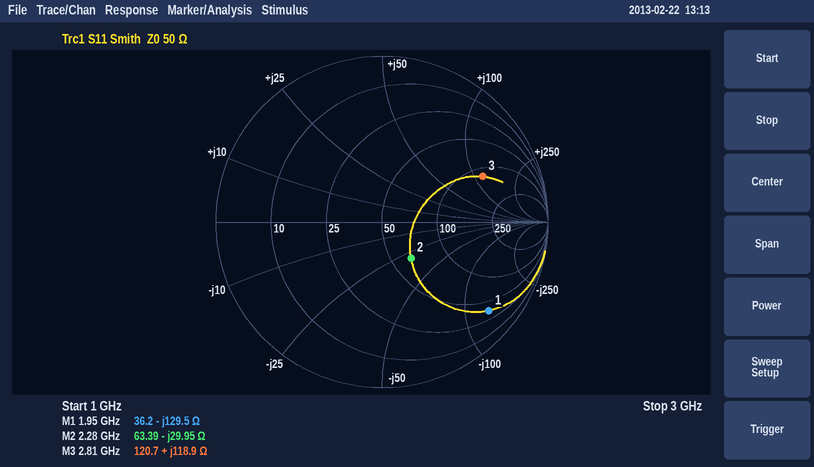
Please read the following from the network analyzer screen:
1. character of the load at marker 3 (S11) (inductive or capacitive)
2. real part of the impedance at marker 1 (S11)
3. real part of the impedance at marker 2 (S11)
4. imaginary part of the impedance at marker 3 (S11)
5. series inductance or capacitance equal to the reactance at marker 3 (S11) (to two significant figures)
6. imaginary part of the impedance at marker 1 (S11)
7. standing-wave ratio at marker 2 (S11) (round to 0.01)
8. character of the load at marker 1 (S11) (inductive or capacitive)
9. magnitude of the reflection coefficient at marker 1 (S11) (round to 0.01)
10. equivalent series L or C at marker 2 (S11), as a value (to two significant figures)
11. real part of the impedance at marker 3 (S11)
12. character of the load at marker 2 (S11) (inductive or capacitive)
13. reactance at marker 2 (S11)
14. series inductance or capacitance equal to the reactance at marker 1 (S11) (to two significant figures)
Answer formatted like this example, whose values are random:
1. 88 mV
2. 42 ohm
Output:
1. inductive
2. 36.2 Ω
3. 63.39 Ω
4. +118.9 Ω
5. 6.7 nH
6. -129.5 Ω
7. 1.78
8. capacitive
9. 0.84
10. 2.3 pF
11. 120.7 Ω
12. capacitive
13. -29.95 Ω
14. 630 fF
